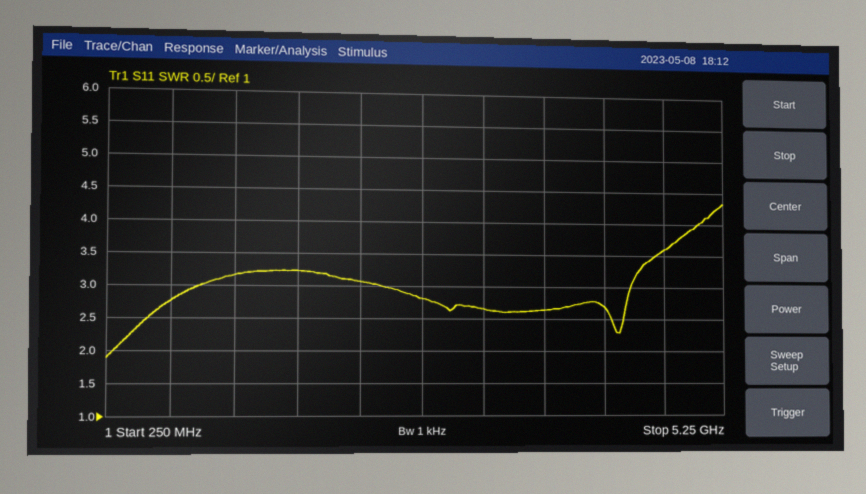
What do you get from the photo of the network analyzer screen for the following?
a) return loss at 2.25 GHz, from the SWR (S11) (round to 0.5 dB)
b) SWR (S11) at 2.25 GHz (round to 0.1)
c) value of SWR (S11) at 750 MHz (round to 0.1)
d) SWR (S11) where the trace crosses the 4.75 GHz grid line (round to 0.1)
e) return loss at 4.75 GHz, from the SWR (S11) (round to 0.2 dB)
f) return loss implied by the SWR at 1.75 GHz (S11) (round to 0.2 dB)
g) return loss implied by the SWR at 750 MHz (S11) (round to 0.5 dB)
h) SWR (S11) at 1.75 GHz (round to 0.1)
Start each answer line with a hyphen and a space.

- 6.0 dB
- 3.1
- 2.8
- 3.6
- 5.0 dB
- 5.6 dB
- 6.5 dB
- 3.2
